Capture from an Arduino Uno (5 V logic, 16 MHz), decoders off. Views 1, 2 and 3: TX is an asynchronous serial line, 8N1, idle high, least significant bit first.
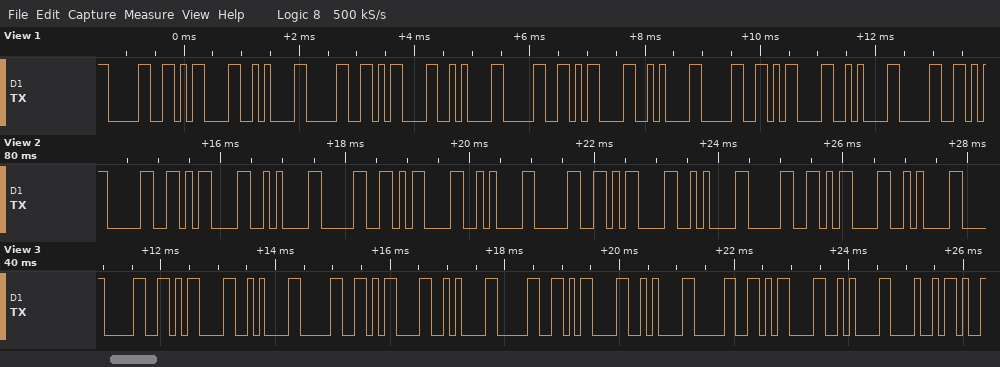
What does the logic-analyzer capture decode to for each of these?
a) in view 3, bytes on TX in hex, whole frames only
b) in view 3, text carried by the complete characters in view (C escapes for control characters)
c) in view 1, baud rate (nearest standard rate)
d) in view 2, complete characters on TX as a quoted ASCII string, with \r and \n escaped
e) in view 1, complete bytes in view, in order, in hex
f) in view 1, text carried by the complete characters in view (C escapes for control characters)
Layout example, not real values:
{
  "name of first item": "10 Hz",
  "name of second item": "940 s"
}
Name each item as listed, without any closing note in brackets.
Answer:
{
  "in view 3, bytes on TX in hex, whole frames only": "30 0D 0A 30 0D 0A 30 0D 0A 30 0D 0A 48",
  "in view 3, text carried by the complete characters in view": "\"0\\r\\n0\\r\\n0\\r\\n0\\r\\nH\"",
  "in view 1, baud rate": "9600 baud",
  "in view 2, complete characters on TX as a quoted ASCII string, with \\r and \\n escaped": "\"0\\r\\n0\\r\\n0\\r\\n0\\r\\n\"",
  "in view 1, complete bytes in view, in order, in hex": "0x30 0x0D 0x0A 0x30 0x0D 0x0A 0x30 0x0D 0x0A 0x30 0x0D 0x0A 0x30",
  "in view 1, text carried by the complete characters in view": "\"0\\r\\n0\\r\\n0\\r\\n0\\r\\n0\""
}
